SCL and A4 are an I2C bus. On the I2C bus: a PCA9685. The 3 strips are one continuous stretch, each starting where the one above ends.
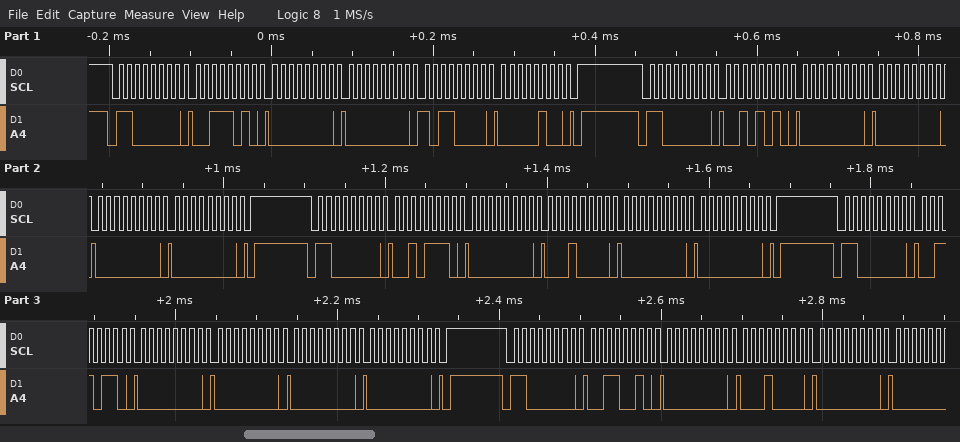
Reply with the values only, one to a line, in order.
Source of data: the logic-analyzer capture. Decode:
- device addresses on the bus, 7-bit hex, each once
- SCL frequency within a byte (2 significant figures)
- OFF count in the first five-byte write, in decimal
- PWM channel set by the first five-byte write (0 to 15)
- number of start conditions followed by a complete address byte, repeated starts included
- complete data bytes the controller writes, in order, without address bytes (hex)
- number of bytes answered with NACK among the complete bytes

0x60
100 kHz
1200
13
5
3A 00 00 B0 04 2A 00 00 00 00 2E 00 10 00 00 36 00 00 00 00 32 00 10 00
0
